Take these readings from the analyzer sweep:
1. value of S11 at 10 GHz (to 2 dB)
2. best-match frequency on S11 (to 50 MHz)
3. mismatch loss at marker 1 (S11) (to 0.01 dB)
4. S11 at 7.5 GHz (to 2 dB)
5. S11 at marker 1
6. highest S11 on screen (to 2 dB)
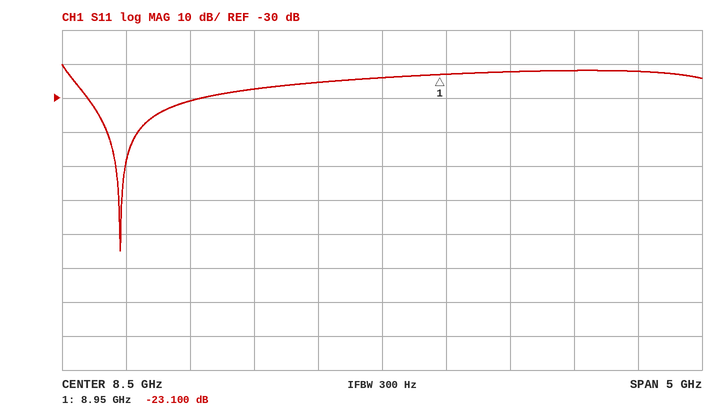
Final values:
-22 dB
6.45 GHz
0.02 dB
-28 dB
-23.100 dB
-20 dB
